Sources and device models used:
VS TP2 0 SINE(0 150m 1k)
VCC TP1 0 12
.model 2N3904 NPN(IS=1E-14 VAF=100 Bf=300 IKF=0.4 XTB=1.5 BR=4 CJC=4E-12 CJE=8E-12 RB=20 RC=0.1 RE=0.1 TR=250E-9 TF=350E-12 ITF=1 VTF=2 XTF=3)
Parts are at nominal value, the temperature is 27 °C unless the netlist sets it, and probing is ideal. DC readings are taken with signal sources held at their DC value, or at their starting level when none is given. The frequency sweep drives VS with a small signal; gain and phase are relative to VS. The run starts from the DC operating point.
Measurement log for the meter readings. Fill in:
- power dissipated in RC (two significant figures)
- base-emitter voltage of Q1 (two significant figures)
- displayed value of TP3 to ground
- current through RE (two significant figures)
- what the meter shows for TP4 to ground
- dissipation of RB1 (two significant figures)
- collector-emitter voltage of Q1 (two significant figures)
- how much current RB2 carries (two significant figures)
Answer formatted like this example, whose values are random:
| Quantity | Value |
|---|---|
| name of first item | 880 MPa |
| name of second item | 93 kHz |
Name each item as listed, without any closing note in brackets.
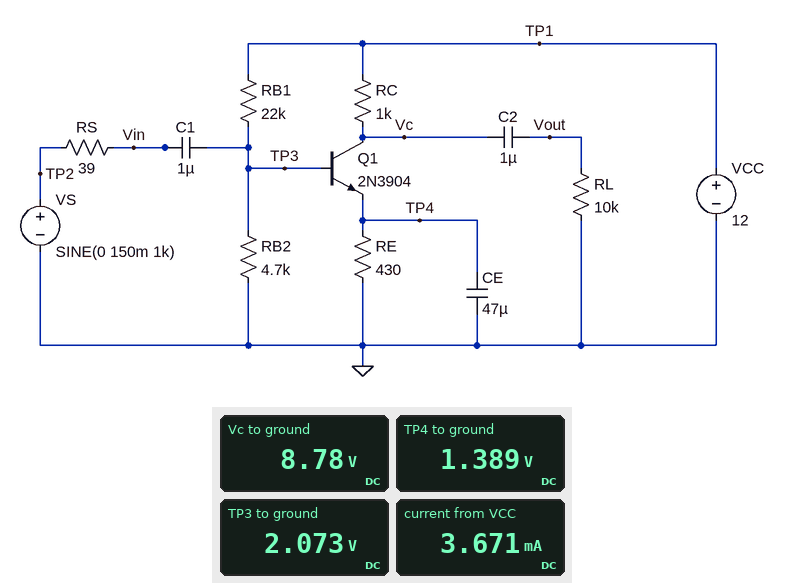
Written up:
| Quantity | Value |
|---|---|
| power dissipated in RC | 10 mW |
| base-emitter voltage of Q1 | 680 mV |
| displayed value of TP3 to ground | 2.073 V |
| current through RE | 3.2 mA |
| what the meter shows for TP4 to ground | 1.389 V |
| dissipation of RB1 | 4.5 mW |
| collector-emitter voltage of Q1 | 7.4 V |
| how much current RB2 carries | 440 µA |
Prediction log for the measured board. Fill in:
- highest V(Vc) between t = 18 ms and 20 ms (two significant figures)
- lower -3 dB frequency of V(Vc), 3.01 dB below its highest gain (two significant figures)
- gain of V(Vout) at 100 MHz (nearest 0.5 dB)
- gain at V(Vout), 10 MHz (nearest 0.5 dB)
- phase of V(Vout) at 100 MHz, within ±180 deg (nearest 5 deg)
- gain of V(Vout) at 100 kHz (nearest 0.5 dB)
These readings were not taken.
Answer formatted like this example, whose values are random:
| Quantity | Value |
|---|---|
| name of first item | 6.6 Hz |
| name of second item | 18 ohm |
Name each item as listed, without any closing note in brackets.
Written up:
| Quantity | Value |
|---|---|
| highest V(Vc) between t = 18 ms and 20 ms | 12 V |
| lower -3 dB frequency of V(Vc), 3.01 dB below its highest gain | 470 Hz |
| gain of V(Vout) at 100 MHz | 20.0 dB |
| gain at V(Vout), 10 MHz | 37.5 dB |
| phase of V(Vout) at 100 MHz, within ±180 deg | 85 deg |
| gain of V(Vout) at 100 kHz | 40.5 dB |
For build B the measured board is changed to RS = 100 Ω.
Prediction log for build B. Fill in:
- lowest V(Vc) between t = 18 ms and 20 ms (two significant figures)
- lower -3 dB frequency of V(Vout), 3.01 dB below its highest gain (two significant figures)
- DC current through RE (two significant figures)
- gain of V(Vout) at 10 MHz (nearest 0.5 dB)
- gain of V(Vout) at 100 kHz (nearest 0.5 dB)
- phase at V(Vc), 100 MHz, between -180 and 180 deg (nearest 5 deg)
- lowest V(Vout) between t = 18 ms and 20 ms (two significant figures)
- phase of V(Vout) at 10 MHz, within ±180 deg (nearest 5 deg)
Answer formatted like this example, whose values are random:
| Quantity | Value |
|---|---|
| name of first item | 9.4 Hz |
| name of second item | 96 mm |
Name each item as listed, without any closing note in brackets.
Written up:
| Quantity | Value |
|---|---|
| lowest V(Vc) between t = 18 ms and 20 ms | 1.5 V |
| lower -3 dB frequency of V(Vout), 3.01 dB below its highest gain | 460 Hz |
| DC current through RE | 3.2 mA |
| gain of V(Vout) at 10 MHz | 33.5 dB |
| gain of V(Vout) at 100 kHz | 40.0 dB |
| phase at V(Vc), 100 MHz, between -180 and 180 deg | 80 deg |
| lowest V(Vout) between t = 18 ms and 20 ms | -7.4 V |
| phase of V(Vout) at 10 MHz, within ±180 deg | 115 deg |
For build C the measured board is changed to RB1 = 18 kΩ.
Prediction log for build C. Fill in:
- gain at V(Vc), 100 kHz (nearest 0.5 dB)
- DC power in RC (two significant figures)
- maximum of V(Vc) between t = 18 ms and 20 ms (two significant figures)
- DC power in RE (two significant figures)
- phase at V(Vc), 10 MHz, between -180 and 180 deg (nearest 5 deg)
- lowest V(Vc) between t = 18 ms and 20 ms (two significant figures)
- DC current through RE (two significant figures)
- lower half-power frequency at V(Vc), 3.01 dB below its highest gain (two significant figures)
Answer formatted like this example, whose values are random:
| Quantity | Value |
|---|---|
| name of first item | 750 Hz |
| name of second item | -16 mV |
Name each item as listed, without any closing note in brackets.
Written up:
| Quantity | Value |
|---|---|
| gain at V(Vc), 100 kHz | 42.0 dB |
| DC power in RC | 16 mW |
| maximum of V(Vc) between t = 18 ms and 20 ms | 12 V |
| DC power in RE | 7.1 mW |
| phase at V(Vc), 10 MHz, between -180 and 180 deg | 125 deg |
| lowest V(Vc) between t = 18 ms and 20 ms | 1.7 V |
| DC current through RE | 4.1 mA |
| lower half-power frequency at V(Vc), 3.01 dB below its highest gain | 580 Hz |
